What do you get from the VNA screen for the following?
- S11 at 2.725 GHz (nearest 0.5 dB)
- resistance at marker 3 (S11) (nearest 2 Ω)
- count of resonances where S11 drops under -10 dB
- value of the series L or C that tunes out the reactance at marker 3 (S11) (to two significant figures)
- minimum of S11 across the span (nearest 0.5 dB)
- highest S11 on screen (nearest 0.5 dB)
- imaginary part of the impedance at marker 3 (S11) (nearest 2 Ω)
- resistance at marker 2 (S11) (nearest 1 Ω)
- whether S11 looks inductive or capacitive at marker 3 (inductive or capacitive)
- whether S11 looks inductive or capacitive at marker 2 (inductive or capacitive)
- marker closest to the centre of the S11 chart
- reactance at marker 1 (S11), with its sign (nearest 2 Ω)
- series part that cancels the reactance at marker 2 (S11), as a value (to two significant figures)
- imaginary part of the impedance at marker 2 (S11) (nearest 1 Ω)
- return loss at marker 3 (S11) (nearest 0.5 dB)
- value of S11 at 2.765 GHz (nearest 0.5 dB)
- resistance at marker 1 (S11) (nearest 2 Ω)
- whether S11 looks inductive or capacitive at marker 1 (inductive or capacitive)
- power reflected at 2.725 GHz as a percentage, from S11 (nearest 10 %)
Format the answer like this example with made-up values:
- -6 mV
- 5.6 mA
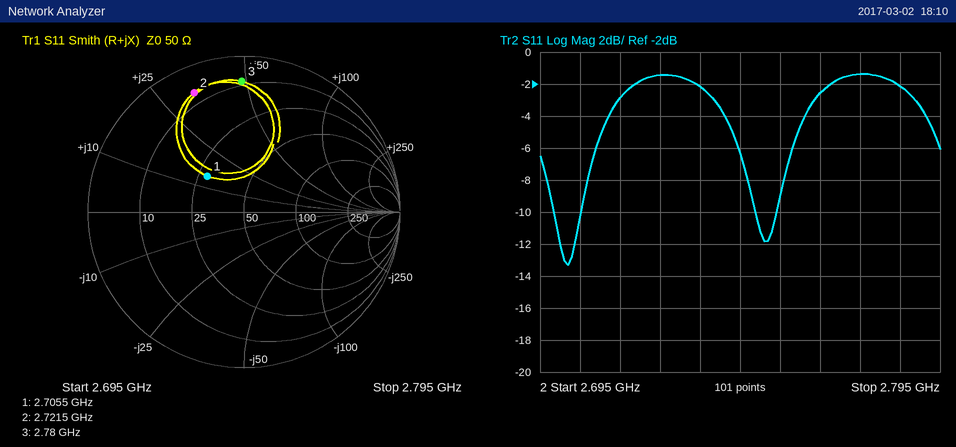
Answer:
- -1.5 dB
- 8 Ω
- 2
- 1.2 pF
- -13.5 dB
- -1.5 dB
- +48 Ω
- 7 Ω
- inductive
- inductive
- marker 1
- +14 Ω
- 1.8 pF
- +33 Ω
- 1.5 dB
- -2.5 dB
- 28 Ω
- inductive
- 70 %
